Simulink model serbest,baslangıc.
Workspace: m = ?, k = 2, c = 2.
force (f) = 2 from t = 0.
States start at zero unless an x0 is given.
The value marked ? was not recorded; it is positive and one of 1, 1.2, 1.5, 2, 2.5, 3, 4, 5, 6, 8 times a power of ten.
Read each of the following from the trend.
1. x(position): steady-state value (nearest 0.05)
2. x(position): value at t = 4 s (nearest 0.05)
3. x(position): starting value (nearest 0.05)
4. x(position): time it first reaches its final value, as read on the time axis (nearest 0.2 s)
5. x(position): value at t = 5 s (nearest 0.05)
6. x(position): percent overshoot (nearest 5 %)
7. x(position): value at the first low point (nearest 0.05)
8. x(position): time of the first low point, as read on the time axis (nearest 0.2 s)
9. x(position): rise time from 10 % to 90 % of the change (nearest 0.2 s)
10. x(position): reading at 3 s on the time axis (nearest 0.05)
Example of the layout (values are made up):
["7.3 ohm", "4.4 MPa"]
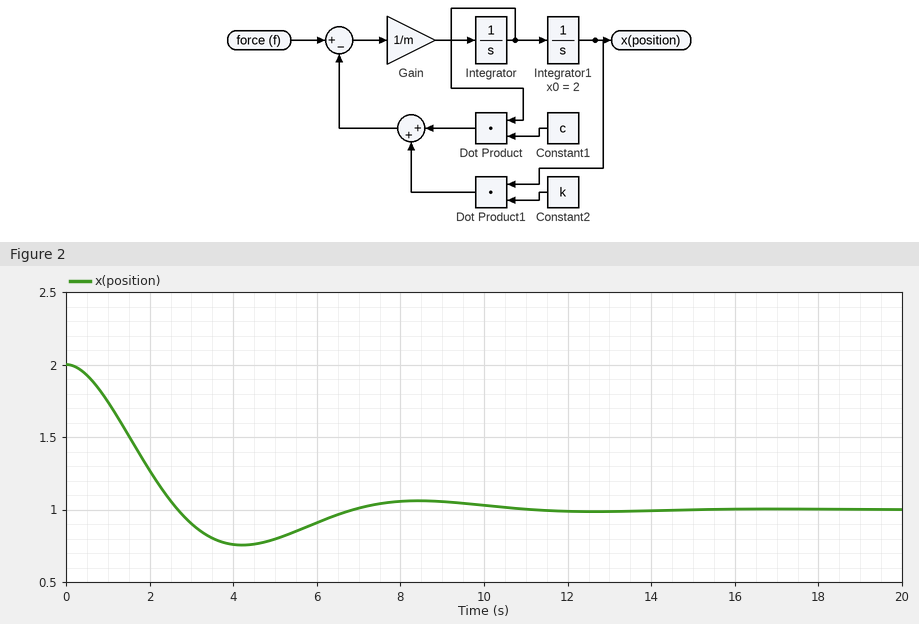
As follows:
["1.00", "0.75", "2.00", "2.6 s", "0.80", "25 %", "0.75", "4.2 s", "1.8 s", "0.90"]
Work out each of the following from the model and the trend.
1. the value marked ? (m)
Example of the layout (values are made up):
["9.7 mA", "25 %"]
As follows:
["3"]
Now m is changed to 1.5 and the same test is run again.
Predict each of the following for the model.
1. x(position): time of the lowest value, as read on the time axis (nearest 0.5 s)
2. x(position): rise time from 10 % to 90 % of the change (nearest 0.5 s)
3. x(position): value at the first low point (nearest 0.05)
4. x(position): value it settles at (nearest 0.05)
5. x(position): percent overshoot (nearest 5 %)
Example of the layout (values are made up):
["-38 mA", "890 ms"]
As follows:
["3.5 s", "1.5 s", "0.90", "1.00", "10 %"]
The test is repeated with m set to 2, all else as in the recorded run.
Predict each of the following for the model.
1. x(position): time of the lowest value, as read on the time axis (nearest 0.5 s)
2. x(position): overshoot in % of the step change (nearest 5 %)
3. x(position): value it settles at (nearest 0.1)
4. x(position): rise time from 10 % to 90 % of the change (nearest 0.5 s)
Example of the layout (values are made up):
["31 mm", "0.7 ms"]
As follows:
["3.5 s", "15 %", "1.0", "1.5 s"]
